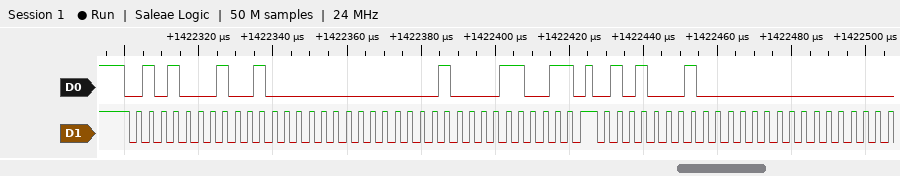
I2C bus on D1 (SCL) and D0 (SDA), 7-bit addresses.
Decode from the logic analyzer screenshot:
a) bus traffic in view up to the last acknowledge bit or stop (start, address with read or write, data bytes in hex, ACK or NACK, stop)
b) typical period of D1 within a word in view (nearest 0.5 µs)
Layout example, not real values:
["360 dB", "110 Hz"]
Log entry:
["start, address 28 read ACK, 40 ACK, 01 ACK, 19 NACK, stop, start, address 28 read ACK, 00 ACK", "3.5 µs"]
